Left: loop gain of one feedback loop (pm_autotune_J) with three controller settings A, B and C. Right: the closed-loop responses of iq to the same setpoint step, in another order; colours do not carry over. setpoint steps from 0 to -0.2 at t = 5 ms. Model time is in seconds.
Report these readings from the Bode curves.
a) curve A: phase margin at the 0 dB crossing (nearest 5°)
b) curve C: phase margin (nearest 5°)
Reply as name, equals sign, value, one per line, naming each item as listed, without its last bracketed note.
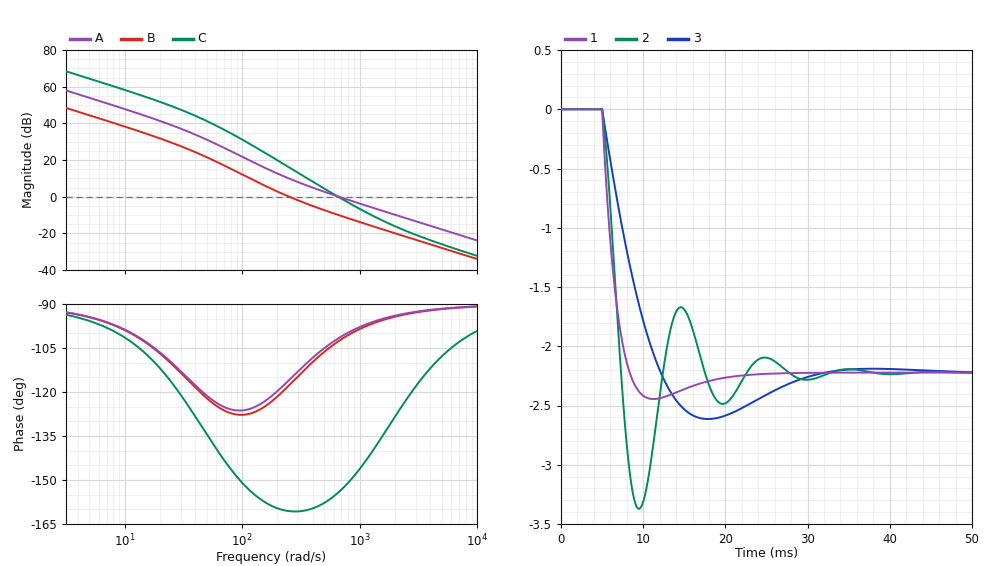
curve A: phase margin at the 0 dB crossing = 80°
curve C: phase margin = 25°
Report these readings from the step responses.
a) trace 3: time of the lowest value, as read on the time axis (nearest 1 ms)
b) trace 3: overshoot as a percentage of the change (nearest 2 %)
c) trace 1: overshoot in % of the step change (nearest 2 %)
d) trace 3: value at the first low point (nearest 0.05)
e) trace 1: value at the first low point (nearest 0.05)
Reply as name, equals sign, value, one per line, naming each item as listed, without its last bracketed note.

trace 3: time of the lowest value, as read on the time axis = 18 ms
trace 3: overshoot as a percentage of the change = 18 %
trace 1: overshoot in % of the step change = 10 %
trace 3: value at the first low point = -2.60
trace 1: value at the first low point = -2.45
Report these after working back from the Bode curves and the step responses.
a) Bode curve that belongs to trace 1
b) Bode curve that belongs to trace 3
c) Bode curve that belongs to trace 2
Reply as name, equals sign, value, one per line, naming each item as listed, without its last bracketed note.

Bode curve that belongs to trace 1 = A
Bode curve that belongs to trace 3 = B
Bode curve that belongs to trace 2 = C
